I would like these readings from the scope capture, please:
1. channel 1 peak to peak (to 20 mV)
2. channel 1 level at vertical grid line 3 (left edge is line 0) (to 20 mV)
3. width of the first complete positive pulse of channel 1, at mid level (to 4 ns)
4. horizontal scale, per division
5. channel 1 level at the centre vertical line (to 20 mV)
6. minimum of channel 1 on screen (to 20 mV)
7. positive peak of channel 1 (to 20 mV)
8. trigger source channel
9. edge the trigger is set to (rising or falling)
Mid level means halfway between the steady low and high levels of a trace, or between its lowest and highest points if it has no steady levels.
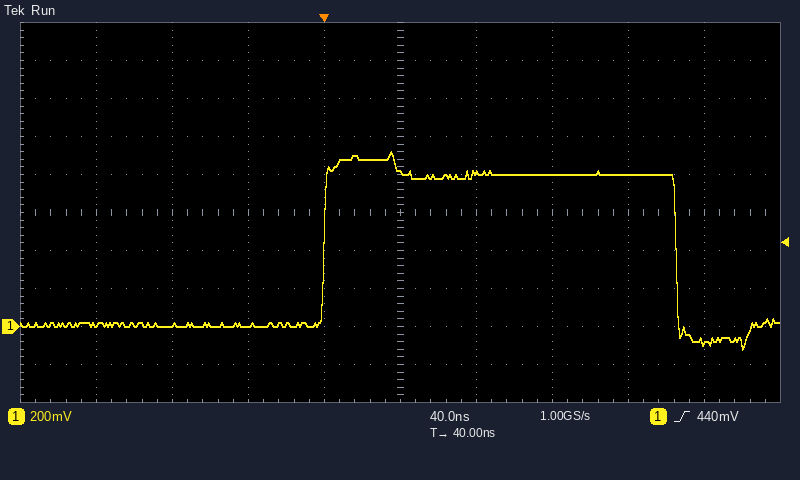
1.04 V
0 mV
184 ns
40 ns
820 mV
-120 mV
920 mV
channel 1
rising
